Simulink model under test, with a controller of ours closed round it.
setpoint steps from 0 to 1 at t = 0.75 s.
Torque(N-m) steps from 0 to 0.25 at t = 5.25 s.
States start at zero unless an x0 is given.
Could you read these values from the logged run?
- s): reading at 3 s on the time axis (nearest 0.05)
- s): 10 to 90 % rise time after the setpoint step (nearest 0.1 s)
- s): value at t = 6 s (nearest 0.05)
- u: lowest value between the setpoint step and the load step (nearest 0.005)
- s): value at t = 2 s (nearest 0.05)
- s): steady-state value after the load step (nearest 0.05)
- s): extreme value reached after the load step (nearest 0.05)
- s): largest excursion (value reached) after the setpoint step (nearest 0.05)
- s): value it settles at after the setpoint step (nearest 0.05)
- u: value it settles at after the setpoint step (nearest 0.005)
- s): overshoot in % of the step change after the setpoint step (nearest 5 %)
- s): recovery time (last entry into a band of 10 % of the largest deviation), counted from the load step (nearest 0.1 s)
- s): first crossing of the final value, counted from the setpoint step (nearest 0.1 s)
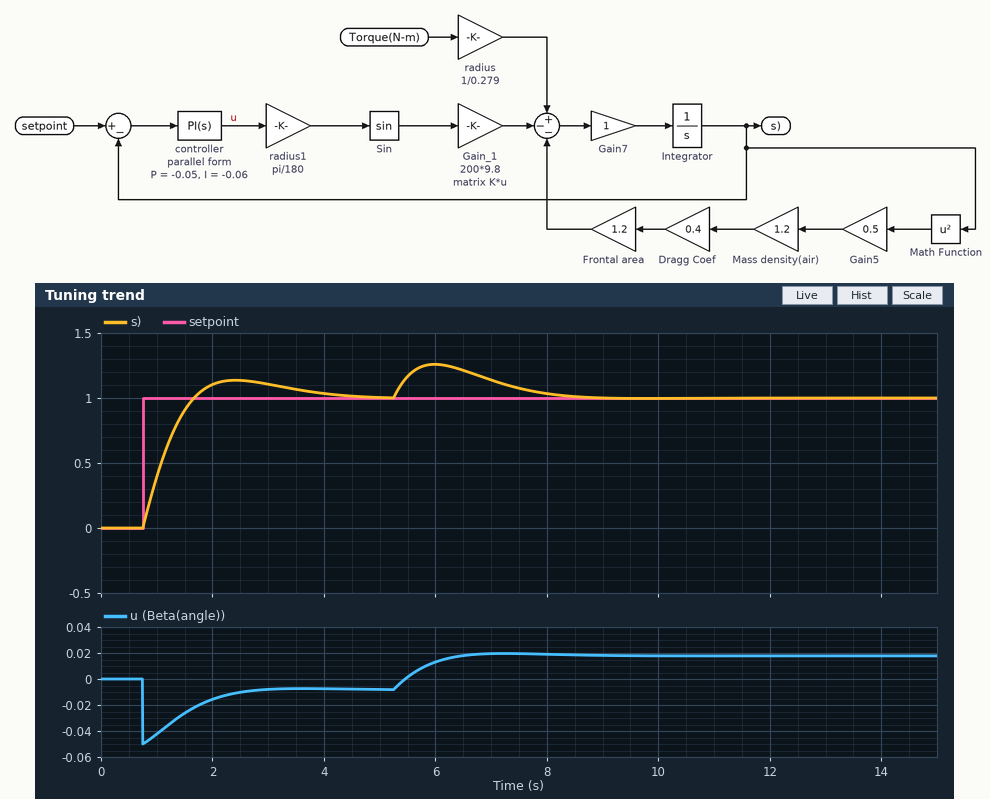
1.10
0.7 s
1.25
-0.050
1.10
1.00
1.25
1.15
1.00
-0.010
15 %
2.9 s
0.9 s
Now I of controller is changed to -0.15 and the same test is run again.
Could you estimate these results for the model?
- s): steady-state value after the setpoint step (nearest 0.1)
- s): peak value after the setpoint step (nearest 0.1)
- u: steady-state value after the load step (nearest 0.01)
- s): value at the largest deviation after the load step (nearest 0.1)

1.0
1.3
0.02
1.2
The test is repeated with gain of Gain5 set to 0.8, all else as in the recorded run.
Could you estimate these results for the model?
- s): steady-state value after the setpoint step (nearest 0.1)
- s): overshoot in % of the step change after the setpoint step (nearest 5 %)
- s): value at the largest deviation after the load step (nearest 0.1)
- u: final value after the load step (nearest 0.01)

1.0
10 %
1.2
0.01
